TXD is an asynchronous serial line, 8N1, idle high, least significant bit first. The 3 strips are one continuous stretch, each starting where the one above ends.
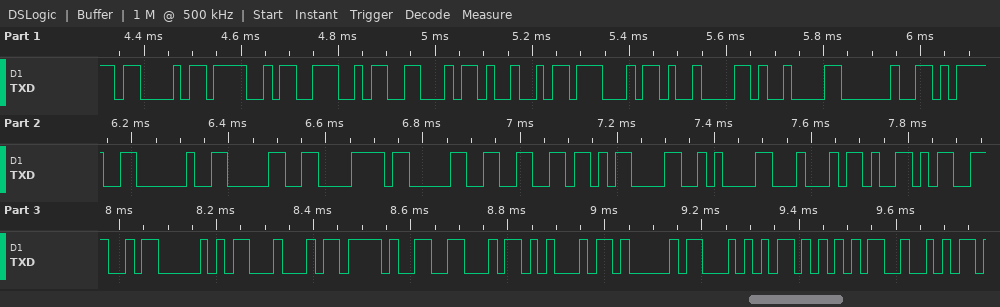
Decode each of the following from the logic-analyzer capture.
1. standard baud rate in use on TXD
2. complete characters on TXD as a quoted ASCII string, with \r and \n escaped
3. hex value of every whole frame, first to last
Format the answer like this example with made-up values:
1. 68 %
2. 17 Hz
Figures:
1. 57600 baud
2. "CONFIG\t\t = 0x0f\r\nDYNPD/FEATUR"
3. 0x43 0x4F 0x4E 0x46 0x49 0x47 0x09 0x09 0x20 0x3D 0x20 0x30 0x78 0x30 0x66 0x0D 0x0A 0x44 0x59 0x4E 0x50 0x44 0x2F 0x46 0x45 0x41 0x54 0x55 0x52
